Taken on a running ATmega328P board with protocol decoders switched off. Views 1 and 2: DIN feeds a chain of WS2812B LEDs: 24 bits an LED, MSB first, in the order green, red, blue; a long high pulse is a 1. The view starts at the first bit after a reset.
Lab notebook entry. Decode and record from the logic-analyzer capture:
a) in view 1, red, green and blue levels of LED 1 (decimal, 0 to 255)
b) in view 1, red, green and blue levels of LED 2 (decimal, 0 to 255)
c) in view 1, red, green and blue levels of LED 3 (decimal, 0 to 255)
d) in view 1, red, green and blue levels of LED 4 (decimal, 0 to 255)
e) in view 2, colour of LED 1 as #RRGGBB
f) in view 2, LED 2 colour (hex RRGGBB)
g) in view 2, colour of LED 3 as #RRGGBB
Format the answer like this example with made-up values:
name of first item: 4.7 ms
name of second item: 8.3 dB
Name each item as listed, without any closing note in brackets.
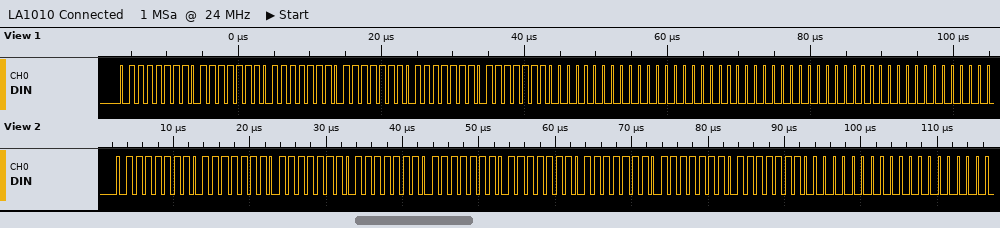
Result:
in view 1, red, green and blue levels of LED 1: 127, 127, 127
in view 1, red, green and blue levels of LED 2: 127, 127, 127
in view 1, red, green and blue levels of LED 3: 0, 0, 0
in view 1, red, green and blue levels of LED 4: 0, 0, 0
in view 2, colour of LED 1 as #RRGGBB: #7F7F7F
in view 2, LED 2 colour: #7F7F7F
in view 2, colour of LED 3 as #RRGGBB: #7F7F7F
